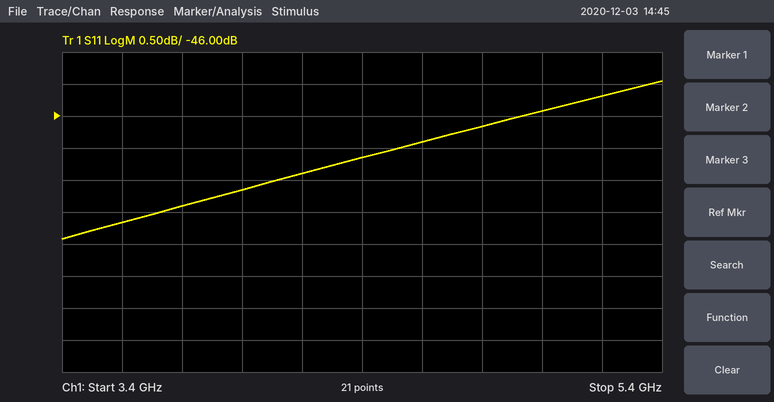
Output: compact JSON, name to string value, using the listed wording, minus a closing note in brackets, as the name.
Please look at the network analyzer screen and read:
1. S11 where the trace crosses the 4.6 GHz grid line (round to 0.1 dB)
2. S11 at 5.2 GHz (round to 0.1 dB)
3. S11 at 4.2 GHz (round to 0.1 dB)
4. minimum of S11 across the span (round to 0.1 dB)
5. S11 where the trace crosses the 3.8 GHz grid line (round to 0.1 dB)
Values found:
{"S11 where the trace crosses the 4.6 GHz grid line": "-46.4 dB", "S11 at 5.2 GHz": "-45.7 dB", "S11 at 4.2 GHz": "-46.9 dB", "minimum of S11 across the span": "-47.9 dB", "S11 where the trace crosses the 3.8 GHz grid line": "-47.4 dB"}
